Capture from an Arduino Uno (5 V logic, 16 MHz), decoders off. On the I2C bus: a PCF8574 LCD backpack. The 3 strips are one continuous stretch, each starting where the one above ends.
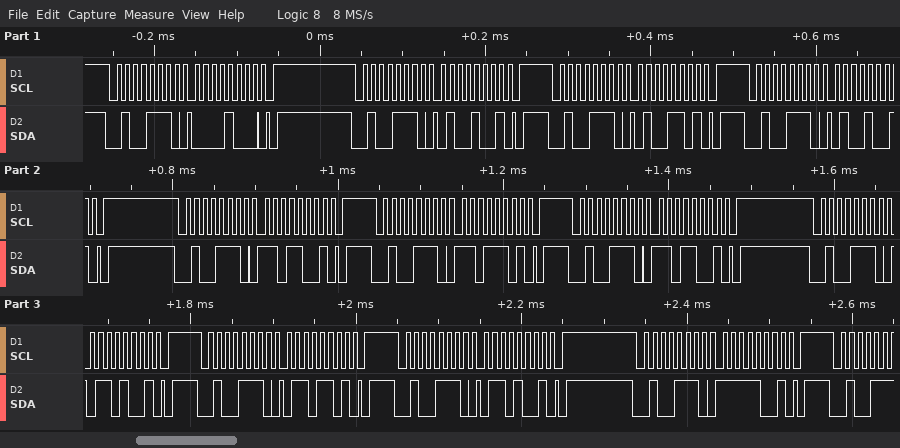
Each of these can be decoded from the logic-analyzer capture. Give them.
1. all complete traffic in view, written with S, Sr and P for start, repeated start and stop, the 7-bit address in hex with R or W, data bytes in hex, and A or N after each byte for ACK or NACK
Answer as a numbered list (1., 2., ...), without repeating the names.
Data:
1. S 27W A 08 A P S 27W A 49 A P S 27W A 4D A P S 27W A 49 A P S 27W A D9 A P S 27W A DD A P S 27W A D9 A P S 27W A 69 A P S 27W A 6D A P S 27W A 69 A P S 27W A F9 A P
